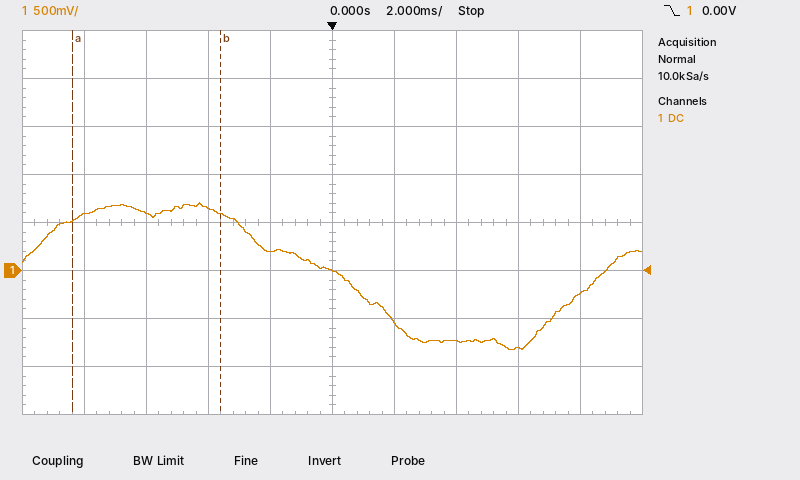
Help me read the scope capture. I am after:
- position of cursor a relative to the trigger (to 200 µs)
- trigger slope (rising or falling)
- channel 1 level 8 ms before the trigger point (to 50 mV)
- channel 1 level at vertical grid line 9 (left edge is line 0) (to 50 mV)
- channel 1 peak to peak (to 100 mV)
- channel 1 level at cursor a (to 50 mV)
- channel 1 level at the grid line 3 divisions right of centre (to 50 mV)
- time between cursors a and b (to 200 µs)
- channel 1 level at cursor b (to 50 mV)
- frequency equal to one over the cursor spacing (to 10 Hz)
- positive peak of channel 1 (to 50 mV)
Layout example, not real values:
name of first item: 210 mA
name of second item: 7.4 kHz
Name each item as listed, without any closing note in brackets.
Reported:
position of cursor a relative to the trigger: -8.4 ms
trigger slope: falling
channel 1 level 8 ms before the trigger point: 600 mV
channel 1 level at vertical grid line 9 (left edge is line 0): -250 mV
channel 1 peak to peak: 1.50 V
channel 1 level at cursor a: 500 mV
channel 1 level at the grid line 3 divisions right of centre: -800 mV
time between cursors a and b: 4.8 ms
channel 1 level at cursor b: 600 mV
frequency equal to one over the cursor spacing: 210 Hz
positive peak of channel 1: 700 mV
